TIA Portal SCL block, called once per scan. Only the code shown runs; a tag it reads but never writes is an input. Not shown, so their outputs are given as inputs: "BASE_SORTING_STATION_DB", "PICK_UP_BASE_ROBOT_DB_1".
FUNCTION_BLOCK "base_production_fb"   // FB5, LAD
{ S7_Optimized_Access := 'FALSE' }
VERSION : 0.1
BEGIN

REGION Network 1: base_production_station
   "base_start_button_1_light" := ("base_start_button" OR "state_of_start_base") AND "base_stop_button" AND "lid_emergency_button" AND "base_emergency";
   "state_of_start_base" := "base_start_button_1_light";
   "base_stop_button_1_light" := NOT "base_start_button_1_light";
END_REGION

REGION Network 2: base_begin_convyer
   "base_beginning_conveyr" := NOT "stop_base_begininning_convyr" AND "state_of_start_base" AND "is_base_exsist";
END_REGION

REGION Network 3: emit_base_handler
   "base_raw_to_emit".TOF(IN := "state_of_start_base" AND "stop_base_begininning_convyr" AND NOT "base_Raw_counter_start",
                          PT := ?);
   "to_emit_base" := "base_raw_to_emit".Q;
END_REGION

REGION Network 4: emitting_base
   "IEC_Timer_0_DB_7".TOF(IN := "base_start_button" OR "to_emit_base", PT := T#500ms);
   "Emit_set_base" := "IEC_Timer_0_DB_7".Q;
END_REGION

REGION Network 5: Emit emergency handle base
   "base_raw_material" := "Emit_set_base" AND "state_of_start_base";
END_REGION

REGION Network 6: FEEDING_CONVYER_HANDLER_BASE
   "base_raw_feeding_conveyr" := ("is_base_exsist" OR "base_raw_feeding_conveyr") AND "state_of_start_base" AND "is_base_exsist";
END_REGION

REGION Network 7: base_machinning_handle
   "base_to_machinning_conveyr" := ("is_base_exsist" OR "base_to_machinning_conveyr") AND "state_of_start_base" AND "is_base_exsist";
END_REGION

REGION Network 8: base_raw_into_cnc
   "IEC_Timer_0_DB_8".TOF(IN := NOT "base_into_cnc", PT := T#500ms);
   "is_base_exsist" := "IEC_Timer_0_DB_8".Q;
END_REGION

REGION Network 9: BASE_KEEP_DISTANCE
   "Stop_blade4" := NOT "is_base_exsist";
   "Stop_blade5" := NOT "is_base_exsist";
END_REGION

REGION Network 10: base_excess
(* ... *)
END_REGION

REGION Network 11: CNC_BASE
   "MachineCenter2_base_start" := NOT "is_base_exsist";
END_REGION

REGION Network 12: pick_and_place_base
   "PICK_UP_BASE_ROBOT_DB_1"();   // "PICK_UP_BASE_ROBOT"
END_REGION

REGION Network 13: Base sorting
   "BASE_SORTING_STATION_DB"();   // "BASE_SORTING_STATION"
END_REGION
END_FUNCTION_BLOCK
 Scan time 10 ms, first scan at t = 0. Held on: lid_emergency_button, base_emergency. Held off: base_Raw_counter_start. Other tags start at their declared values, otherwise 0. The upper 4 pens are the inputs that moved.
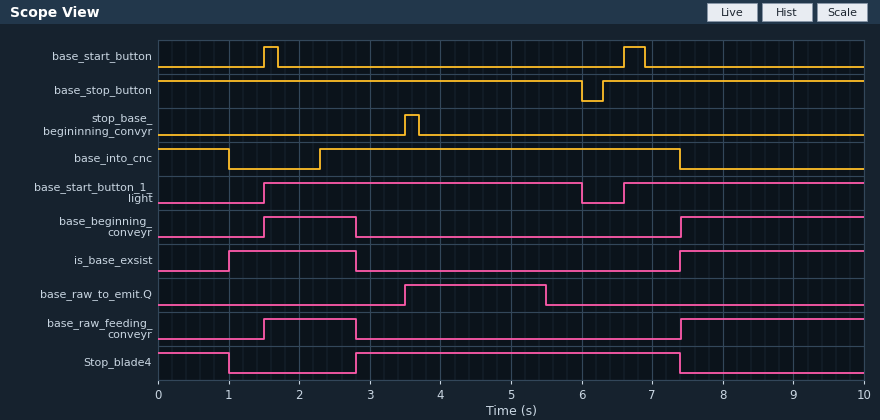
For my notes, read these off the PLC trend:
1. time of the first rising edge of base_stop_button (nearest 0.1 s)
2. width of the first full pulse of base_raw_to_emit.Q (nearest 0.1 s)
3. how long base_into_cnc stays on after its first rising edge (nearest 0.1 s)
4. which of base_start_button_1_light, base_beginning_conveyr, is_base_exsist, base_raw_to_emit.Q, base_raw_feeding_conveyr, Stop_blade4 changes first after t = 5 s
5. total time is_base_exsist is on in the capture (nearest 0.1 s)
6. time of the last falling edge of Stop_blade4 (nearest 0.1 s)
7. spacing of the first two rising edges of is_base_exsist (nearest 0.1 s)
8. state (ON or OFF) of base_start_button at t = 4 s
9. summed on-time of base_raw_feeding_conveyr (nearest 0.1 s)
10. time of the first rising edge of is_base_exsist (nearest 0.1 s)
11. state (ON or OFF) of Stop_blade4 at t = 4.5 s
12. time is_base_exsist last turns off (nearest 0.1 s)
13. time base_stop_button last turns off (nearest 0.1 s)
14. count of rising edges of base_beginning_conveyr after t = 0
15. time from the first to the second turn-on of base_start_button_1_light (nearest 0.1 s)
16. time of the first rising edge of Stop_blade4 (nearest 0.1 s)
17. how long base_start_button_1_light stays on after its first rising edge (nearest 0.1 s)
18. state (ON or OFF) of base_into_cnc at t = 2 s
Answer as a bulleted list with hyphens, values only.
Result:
- 6.3 s
- 2.0 s
- 5.1 s
- base_raw_to_emit.Q
- 4.4 s
- 7.4 s
- 6.4 s
- OFF
- 3.9 s
- 1.0 s
- ON
- 2.8 s
- 6.0 s
- 2
- 5.1 s
- 2.8 s
- 4.5 s
- OFF
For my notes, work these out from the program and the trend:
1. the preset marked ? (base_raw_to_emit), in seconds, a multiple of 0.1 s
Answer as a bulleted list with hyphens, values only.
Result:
- 1.8 s
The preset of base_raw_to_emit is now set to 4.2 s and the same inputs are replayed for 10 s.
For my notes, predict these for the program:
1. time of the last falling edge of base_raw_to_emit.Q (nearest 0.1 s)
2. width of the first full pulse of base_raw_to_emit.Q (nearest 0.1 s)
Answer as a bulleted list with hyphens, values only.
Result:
- 7.9 s
- 4.4 s
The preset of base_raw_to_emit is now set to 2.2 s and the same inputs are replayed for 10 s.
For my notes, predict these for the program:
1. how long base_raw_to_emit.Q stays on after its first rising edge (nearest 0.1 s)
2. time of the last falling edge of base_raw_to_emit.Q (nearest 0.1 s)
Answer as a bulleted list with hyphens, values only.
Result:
- 2.4 s
- 5.9 s
